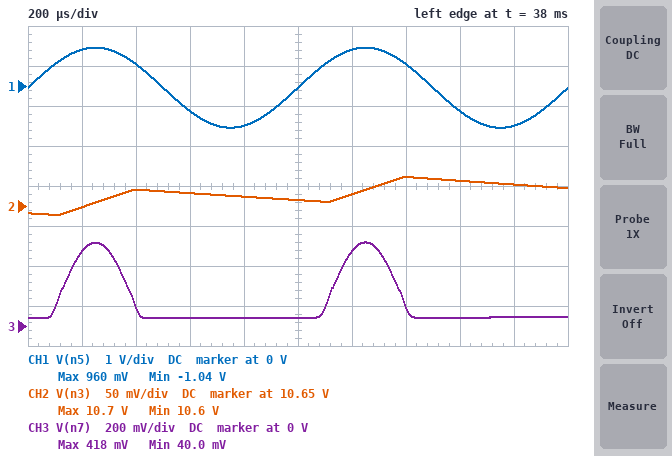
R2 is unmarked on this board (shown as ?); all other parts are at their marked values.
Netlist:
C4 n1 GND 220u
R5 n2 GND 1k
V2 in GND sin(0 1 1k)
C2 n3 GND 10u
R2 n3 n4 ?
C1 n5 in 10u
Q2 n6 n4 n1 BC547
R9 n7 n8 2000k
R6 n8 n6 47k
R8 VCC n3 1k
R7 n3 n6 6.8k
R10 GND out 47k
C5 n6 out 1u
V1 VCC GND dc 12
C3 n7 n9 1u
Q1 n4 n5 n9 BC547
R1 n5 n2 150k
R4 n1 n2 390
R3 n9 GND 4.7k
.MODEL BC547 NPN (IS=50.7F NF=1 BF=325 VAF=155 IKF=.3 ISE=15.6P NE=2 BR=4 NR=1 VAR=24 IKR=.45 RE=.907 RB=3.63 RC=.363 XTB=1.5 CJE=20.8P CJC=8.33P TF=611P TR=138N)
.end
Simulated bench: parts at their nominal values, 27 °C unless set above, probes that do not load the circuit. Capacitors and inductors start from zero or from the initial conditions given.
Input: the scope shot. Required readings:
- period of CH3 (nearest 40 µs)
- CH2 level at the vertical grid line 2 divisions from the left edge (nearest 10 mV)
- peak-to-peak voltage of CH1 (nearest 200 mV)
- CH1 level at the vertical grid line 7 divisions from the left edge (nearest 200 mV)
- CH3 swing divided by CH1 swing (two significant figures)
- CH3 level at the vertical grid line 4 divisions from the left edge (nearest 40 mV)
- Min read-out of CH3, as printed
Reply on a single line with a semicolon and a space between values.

1.00 ms; 10.67 V; 2.0 V; 600 mV; 0.19; 40 mV; 40.0 mV
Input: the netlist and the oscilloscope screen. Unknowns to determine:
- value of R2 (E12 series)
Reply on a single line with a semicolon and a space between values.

470 kΩ
